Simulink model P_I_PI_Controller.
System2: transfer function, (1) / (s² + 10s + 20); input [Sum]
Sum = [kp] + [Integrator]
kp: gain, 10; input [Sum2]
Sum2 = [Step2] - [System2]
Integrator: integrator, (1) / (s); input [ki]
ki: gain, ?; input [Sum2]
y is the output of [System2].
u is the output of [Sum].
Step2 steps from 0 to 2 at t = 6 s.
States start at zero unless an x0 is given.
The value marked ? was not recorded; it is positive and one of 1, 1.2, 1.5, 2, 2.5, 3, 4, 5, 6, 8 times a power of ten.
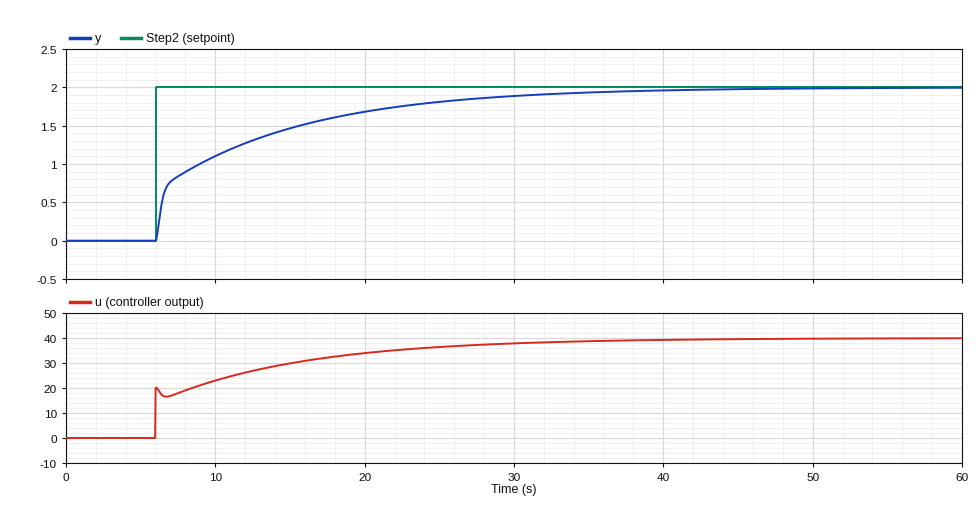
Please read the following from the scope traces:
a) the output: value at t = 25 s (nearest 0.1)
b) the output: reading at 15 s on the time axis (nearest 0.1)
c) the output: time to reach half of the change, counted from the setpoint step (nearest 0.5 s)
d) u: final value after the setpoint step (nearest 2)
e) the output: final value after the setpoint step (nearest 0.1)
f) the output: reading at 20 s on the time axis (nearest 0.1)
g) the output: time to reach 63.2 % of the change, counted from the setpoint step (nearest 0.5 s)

1.8
1.5
3.0 s
40
2.0
1.7
6.0 s
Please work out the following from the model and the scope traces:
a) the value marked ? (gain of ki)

3
